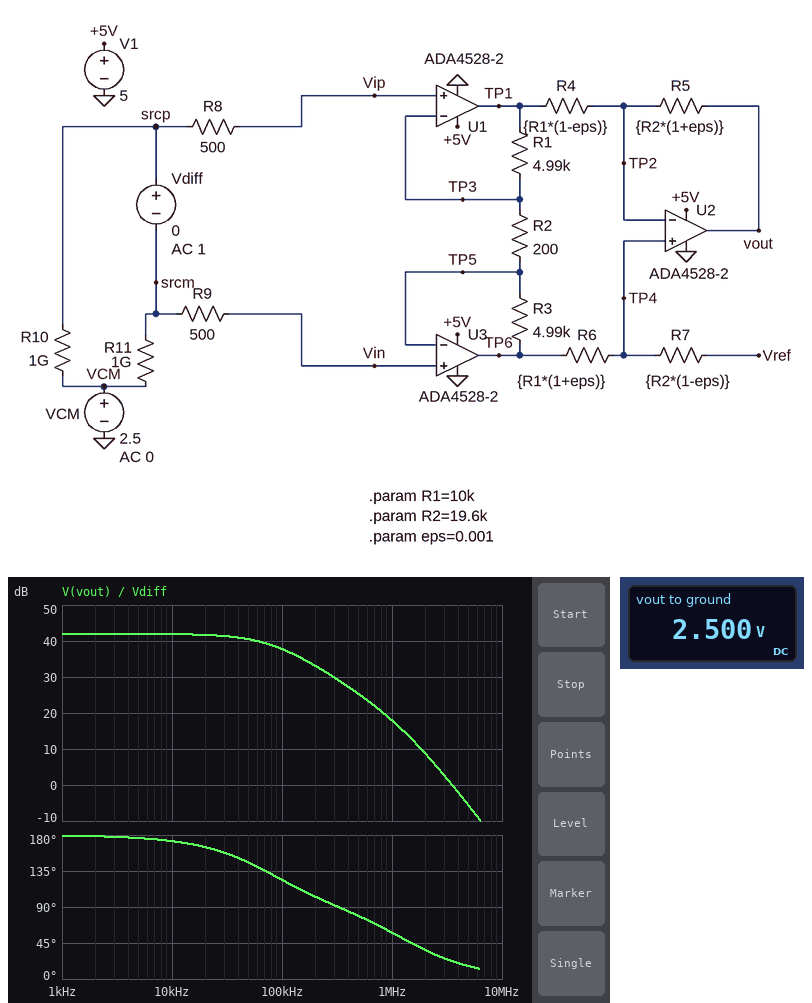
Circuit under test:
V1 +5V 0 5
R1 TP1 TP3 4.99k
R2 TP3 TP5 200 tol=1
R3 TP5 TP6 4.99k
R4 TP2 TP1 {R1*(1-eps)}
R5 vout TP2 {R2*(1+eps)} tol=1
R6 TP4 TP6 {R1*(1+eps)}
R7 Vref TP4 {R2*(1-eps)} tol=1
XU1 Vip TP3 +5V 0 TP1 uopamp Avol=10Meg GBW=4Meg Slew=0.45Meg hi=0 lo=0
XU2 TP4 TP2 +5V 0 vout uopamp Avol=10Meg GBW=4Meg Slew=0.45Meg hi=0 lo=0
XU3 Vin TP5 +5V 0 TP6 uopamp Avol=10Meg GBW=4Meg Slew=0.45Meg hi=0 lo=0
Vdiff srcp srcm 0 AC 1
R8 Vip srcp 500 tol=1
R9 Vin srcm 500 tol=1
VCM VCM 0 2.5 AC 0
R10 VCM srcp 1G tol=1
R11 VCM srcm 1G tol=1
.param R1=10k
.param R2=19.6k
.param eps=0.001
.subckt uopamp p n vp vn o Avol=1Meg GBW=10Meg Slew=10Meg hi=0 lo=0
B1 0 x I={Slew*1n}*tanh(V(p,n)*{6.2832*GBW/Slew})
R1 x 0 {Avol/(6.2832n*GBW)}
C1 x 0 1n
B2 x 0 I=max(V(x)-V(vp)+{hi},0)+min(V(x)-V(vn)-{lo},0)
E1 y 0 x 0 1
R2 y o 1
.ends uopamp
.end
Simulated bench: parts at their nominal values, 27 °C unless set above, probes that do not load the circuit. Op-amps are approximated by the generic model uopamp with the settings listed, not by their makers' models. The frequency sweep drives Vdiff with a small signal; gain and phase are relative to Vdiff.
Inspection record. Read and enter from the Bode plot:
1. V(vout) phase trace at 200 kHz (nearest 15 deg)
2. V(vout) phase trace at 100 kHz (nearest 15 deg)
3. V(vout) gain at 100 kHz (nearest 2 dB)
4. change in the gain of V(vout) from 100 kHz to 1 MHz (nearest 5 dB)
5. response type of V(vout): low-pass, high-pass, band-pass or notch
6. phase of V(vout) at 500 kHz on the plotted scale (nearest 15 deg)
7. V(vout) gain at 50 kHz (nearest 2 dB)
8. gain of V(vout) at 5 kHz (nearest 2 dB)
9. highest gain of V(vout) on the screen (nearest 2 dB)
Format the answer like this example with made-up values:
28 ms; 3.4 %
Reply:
105 deg; 120 deg; 38 dB; -20 dB; low-pass; 75 deg; 40 dB; 42 dB; 42 dB
